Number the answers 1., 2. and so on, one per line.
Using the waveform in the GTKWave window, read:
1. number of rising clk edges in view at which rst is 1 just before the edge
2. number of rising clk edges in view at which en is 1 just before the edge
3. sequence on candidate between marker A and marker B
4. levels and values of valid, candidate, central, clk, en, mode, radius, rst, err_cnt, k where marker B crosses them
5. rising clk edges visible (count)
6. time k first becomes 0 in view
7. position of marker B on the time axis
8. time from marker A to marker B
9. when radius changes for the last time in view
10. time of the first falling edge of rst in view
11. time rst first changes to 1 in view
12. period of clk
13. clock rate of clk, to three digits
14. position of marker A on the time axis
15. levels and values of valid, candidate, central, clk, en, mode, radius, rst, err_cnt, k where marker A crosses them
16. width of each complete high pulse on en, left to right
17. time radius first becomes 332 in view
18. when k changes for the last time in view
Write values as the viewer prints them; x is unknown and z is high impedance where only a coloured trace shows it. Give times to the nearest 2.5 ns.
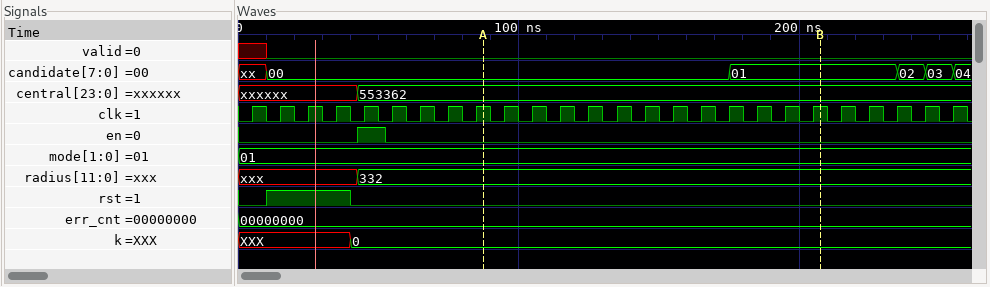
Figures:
1. 3
2. 1
3. 00, 01
4. valid=0, candidate=01, central=553362, clk=1, en=0, mode=01, radius=332, rst=0, err_cnt=00000000, k=0
5. 26
6. 40 ns
7. 207.5 ns
8. 120 ns
9. 42.5 ns
10. 40 ns
11. 10 ns
12. 10 ns
13. 100 MHz
14. 87.5 ns
15. valid=0, candidate=00, central=553362, clk=1, en=0, mode=01, radius=332, rst=0, err_cnt=00000000, k=0
16. 10 ns
17. 42.5 ns
18. 40 ns
